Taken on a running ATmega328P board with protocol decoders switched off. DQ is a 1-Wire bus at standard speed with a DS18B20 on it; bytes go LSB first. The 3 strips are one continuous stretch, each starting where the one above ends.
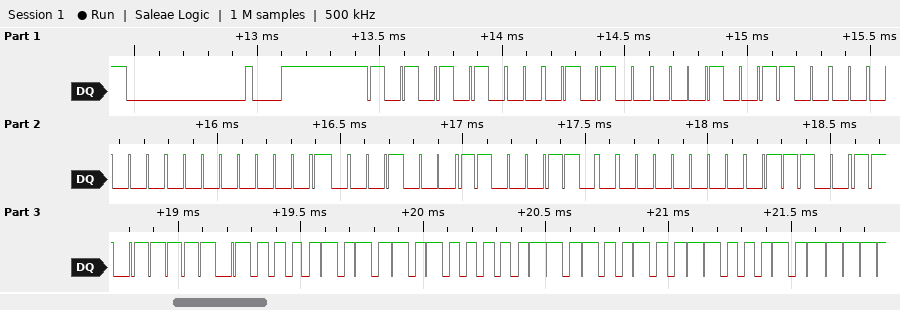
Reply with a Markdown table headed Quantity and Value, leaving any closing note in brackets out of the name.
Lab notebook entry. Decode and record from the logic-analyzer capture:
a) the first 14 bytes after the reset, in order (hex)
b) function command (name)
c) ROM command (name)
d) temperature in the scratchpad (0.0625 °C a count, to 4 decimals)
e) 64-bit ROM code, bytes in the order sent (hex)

| Quantity | Value |
|---|---|
| the first 14 bytes after the reset, in order | 55 28 C8 00 00 11 63 00 CE BE 50 05 4B 46 |
| function command | Read Scratchpad |
| ROM command | Match ROM |
| temperature in the scratchpad | 85.0000 °C |
| 64-bit ROM code, bytes in the order sent | 28 C8 00 00 11 63 00 CE |
